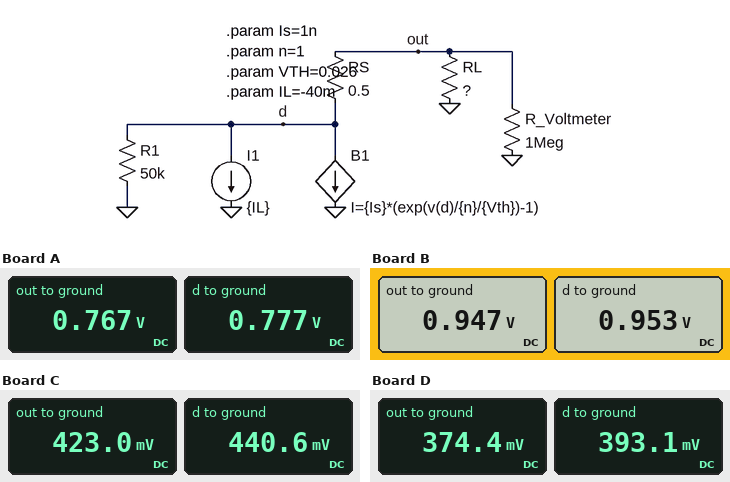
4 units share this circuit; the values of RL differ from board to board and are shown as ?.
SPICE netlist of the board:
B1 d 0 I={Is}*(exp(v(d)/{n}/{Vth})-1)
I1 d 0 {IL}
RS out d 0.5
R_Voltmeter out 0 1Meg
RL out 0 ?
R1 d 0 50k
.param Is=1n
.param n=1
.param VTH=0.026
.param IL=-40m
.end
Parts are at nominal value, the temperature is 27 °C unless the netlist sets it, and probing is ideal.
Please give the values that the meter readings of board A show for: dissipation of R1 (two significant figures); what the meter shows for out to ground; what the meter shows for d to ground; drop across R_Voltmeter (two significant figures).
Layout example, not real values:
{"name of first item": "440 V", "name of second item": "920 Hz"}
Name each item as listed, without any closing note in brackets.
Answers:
{"dissipation of R1": "12 µW", "what the meter shows for out to ground": "0.767 V", "what the meter shows for d to ground": "0.777 V", "drop across R_Voltmeter": "770 mV"}
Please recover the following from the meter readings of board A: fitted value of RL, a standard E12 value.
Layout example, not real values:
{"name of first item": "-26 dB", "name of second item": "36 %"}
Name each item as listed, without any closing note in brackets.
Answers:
{"fitted value of RL, a standard E12 value": "39 Ω"}
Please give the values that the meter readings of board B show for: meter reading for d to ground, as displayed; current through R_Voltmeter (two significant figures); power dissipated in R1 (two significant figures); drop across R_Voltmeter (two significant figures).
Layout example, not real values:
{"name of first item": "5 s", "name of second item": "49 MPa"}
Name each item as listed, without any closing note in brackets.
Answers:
{"meter reading for d to ground, as displayed": "0.953 V", "current through R_Voltmeter": "950 nA", "power dissipated in R1": "18 µW", "drop across R_Voltmeter": "950 mV"}
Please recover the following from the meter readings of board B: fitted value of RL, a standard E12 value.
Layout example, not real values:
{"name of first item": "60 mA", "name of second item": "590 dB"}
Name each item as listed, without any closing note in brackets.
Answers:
{"fitted value of RL, a standard E12 value": "82 Ω"}
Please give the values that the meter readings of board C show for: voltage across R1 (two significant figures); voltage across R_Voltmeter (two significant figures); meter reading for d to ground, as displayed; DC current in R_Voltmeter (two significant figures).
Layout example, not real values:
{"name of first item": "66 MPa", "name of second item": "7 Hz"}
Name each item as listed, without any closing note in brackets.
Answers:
{"voltage across R1": "440 mV", "voltage across R_Voltmeter": "420 mV", "meter reading for d to ground, as displayed": "440.6 mV", "DC current in R_Voltmeter": "420 nA"}
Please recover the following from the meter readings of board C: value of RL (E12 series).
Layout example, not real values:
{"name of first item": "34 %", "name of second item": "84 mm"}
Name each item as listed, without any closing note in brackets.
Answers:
{"value of RL": "12 Ω"}
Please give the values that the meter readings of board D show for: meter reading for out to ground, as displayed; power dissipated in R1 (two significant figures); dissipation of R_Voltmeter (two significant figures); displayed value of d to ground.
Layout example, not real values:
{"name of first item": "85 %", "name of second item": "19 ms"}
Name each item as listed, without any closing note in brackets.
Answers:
{"meter reading for out to ground, as displayed": "374.4 mV", "power dissipated in R1": "3.1 µW", "dissipation of R_Voltmeter": "140 nW", "displayed value of d to ground": "393.1 mV"}
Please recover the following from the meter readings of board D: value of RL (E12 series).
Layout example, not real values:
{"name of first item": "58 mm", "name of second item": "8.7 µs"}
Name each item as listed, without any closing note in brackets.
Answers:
{"value of RL": "10 Ω"}
